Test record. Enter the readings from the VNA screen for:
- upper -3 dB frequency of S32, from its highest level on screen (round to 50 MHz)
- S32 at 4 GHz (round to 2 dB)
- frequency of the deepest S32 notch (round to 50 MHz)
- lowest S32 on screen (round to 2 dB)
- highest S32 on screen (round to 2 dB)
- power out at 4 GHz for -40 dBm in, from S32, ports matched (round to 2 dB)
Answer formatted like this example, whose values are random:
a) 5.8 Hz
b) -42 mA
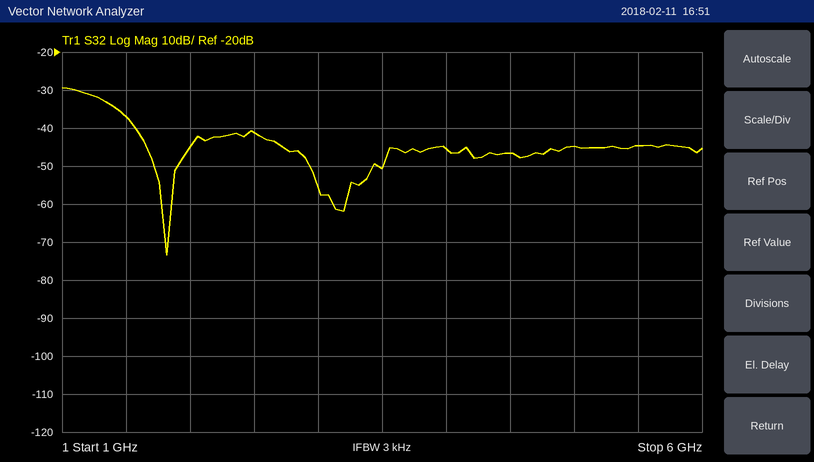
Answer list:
a) 1.30 GHz
b) -46 dB
c) 1.80 GHz
d) -74 dB
e) -30 dB
f) -86 dBm
